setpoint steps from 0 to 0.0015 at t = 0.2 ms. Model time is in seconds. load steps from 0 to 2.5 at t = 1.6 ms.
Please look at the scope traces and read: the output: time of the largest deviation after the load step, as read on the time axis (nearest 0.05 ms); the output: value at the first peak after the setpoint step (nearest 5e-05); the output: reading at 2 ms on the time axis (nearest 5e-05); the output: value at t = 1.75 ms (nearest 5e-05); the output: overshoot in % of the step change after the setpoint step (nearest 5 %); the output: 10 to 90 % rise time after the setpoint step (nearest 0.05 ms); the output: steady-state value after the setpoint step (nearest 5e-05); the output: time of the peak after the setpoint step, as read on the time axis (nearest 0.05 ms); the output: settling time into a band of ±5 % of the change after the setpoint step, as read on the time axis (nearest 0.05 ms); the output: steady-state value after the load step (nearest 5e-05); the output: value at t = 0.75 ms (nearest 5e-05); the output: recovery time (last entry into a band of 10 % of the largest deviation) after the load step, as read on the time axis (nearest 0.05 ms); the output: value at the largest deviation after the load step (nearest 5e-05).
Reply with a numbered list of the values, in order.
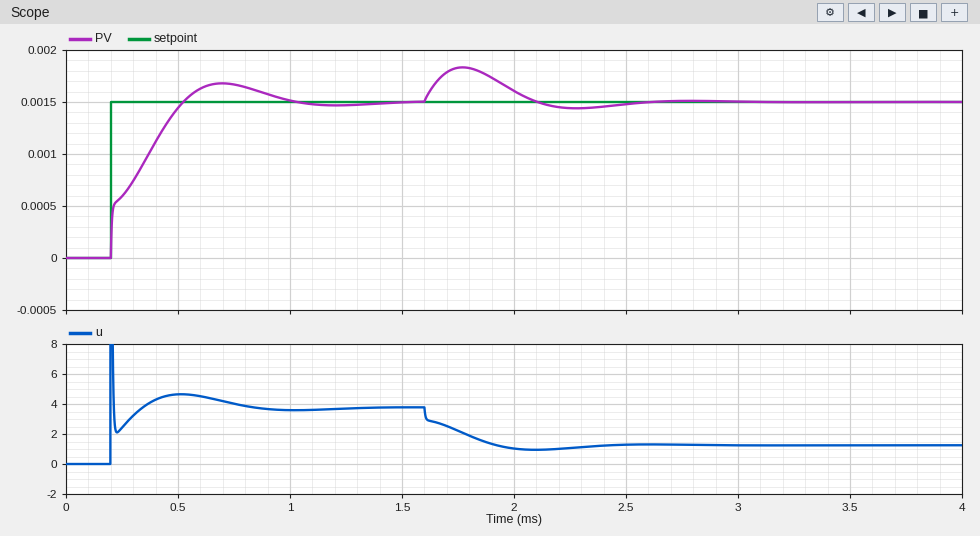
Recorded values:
1. 1.75 ms
2. 0.00170
3. 0.00160
4. 0.00185
5. 10 %
6. 0.25 ms
7. 0.00150
8. 0.70 ms
9. 0.90 ms
10. 0.00150
11. 0.00165
12. 2.45 ms
13. 0.00185
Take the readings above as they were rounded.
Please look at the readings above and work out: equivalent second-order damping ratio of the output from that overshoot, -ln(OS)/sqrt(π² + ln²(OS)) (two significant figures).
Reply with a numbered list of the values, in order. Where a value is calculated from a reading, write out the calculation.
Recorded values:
1. ln(0.1) = -2.303; 2.303 / sqrt(9.870 + 5.302) = 0.59
